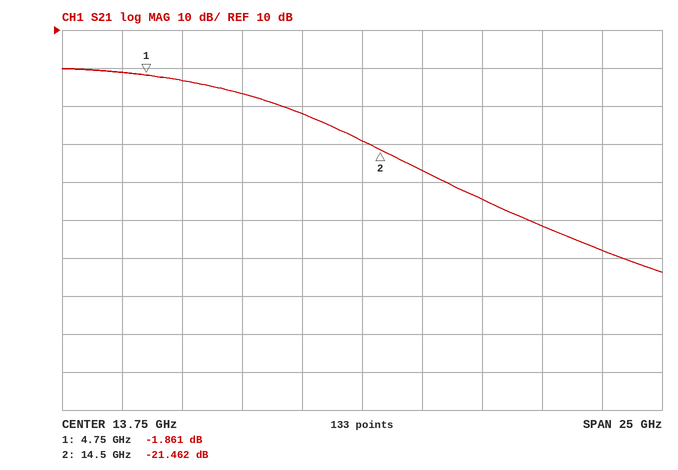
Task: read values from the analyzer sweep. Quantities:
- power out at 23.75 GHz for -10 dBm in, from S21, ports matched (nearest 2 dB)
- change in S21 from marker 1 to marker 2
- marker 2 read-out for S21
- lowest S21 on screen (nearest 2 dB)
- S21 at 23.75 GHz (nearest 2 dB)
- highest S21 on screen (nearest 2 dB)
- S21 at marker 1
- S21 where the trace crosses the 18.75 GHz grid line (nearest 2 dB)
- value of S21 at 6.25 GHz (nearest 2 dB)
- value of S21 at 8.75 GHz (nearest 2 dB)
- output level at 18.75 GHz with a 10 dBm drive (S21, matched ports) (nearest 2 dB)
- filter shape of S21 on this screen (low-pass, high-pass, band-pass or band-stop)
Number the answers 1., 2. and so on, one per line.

1. -58 dBm
2. -19.601 dB
3. -21.462 dB
4. -54 dB
5. -48 dB
6. 0 dB
7. -1.861 dB
8. -34 dB
9. -4 dB
10. -6 dB
11. -24 dBm
12. low-pass
